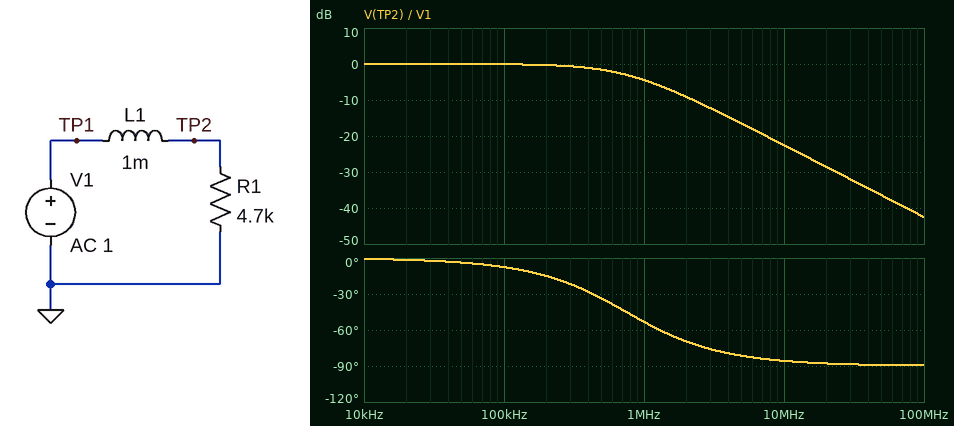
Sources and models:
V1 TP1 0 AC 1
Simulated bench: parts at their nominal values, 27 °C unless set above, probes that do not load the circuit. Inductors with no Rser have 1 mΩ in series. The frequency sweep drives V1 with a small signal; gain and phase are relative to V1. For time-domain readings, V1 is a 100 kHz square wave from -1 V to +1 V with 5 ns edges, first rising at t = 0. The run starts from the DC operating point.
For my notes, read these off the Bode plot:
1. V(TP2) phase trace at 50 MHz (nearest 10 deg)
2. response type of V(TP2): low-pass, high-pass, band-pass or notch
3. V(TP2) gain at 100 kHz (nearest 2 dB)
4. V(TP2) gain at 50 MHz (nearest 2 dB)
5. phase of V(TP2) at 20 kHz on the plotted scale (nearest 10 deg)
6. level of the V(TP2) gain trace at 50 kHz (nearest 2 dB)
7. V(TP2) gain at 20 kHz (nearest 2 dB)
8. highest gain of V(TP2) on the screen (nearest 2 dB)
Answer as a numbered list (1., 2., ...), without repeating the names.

1. -90 deg
2. low-pass
3. 0 dB
4. -36 dB
5. 0 deg
6. 0 dB
7. 0 dB
8. 0 dB
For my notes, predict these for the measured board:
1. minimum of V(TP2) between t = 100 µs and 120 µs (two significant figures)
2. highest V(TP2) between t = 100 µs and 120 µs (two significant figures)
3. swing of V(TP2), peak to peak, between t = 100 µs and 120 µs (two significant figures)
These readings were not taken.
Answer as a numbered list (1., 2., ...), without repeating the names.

1. -1.0 V
2. 1.0 V
3. 2.0 V
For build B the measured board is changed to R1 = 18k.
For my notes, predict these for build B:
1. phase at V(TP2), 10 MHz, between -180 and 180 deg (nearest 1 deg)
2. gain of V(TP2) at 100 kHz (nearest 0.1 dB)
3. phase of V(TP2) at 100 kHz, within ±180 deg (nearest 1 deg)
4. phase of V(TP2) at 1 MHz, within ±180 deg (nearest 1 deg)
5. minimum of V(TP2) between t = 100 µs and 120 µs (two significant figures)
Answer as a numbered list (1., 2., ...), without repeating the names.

1. -74 deg
2. 0 dB
3. -2 deg
4. -19 deg
5. -1.0 V
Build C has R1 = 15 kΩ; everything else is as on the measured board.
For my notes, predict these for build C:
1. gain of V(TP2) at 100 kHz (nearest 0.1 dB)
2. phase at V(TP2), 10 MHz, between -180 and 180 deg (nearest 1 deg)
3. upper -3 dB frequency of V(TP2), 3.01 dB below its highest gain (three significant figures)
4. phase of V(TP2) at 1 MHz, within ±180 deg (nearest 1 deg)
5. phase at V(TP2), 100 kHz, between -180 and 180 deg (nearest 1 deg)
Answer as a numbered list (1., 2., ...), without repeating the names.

1. 0 dB
2. -77 deg
3. 2.39 MHz
4. -23 deg
5. -2 deg
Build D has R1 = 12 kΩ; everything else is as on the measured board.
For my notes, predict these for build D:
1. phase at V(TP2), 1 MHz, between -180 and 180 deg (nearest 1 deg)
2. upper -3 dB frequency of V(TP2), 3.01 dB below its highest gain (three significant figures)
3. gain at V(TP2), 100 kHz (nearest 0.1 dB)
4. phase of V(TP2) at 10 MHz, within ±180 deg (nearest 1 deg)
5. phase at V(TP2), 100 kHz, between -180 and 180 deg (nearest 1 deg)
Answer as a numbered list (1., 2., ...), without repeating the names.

1. -28 deg
2. 1.91 MHz
3. 0 dB
4. -79 deg
5. -3 deg
